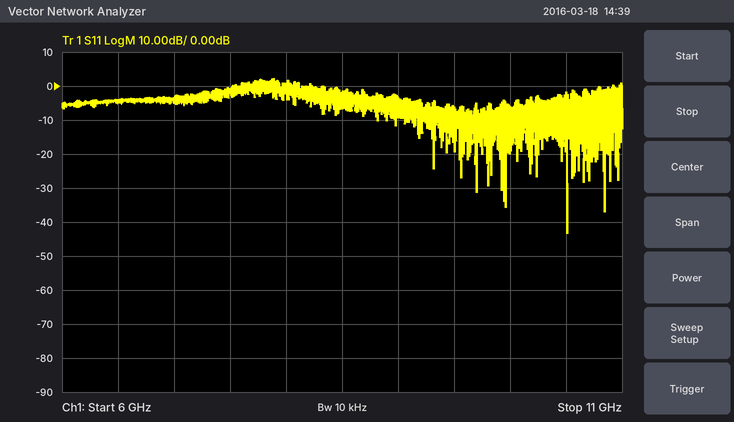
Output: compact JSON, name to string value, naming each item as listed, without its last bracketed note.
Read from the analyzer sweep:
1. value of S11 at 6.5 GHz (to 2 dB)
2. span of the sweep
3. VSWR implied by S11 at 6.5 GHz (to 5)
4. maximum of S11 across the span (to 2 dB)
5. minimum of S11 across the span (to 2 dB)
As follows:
{"value of S11 at 6.5 GHz": "-4 dB", "span of the sweep": "5 GHz", "VSWR implied by S11 at 6.5 GHz": "5", "maximum of S11 across the span": "2 dB", "minimum of S11 across the span": "-44 dB"}
